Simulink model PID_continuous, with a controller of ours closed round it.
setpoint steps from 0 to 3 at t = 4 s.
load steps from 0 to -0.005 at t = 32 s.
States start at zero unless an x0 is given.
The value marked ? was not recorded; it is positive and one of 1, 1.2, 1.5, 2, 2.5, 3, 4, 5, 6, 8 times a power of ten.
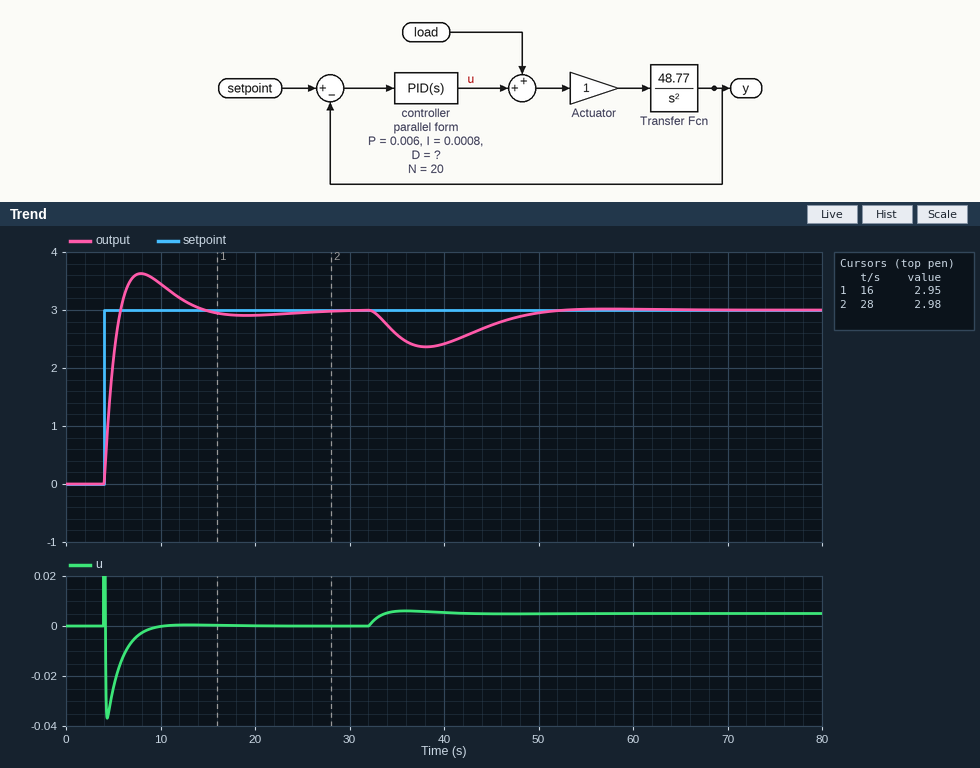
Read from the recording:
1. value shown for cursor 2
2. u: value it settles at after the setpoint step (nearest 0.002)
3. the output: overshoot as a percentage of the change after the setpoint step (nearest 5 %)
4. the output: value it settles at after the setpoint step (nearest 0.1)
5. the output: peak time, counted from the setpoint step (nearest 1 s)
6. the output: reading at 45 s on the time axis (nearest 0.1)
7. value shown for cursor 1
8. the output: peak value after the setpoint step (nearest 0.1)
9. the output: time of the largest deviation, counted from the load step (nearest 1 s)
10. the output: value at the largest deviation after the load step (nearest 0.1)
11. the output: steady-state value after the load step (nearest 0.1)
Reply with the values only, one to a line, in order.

2.98
0.000
20 %
3.0
4 s
2.7
2.95
3.6
6 s
2.4
3.0
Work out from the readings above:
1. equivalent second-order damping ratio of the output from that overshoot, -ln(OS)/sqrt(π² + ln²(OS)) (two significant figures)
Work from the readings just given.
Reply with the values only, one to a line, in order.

0.46
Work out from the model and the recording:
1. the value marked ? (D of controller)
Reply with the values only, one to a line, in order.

0.02
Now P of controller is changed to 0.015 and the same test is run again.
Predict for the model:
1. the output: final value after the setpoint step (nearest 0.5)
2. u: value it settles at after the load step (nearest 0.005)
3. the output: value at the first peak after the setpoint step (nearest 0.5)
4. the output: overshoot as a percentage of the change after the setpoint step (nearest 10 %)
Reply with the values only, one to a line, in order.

3.0
0.005
4.0
30 %
